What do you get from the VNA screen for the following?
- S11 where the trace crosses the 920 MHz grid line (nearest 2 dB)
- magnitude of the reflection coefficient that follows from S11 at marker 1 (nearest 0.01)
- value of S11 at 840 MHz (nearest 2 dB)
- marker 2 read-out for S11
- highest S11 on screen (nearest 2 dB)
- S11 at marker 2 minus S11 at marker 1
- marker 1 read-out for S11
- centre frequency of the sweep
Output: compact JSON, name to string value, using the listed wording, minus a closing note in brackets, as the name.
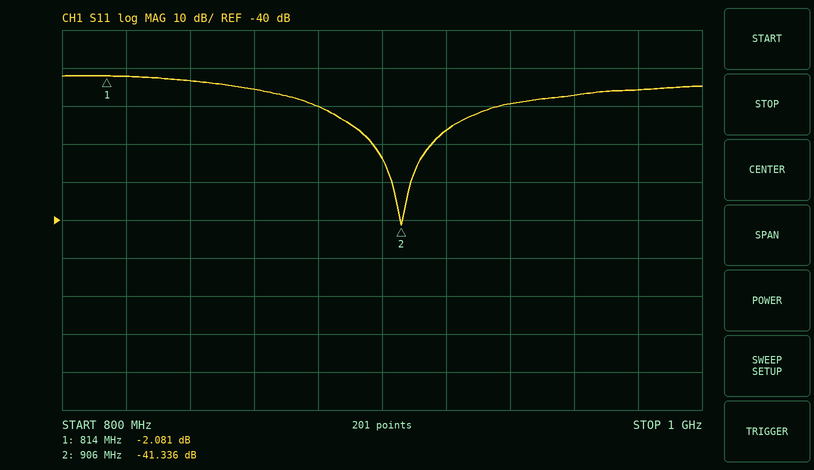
{"S11 where the trace crosses the 920 MHz grid line": "-16 dB", "magnitude of the reflection coefficient that follows from S11 at marker 1": "0.79", "value of S11 at 840 MHz": "-4 dB", "marker 2 read-out for S11": "-41.336 dB", "highest S11 on screen": "-2 dB", "S11 at marker 2 minus S11 at marker 1": "-39.255 dB", "marker 1 read-out for S11": "-2.081 dB", "centre frequency of the sweep": "900 MHz"}
